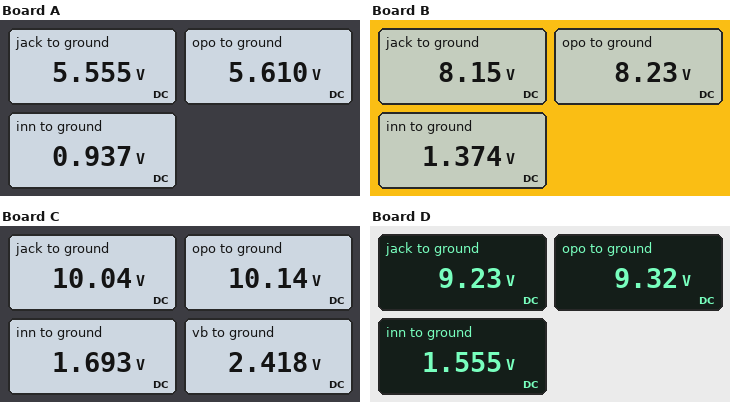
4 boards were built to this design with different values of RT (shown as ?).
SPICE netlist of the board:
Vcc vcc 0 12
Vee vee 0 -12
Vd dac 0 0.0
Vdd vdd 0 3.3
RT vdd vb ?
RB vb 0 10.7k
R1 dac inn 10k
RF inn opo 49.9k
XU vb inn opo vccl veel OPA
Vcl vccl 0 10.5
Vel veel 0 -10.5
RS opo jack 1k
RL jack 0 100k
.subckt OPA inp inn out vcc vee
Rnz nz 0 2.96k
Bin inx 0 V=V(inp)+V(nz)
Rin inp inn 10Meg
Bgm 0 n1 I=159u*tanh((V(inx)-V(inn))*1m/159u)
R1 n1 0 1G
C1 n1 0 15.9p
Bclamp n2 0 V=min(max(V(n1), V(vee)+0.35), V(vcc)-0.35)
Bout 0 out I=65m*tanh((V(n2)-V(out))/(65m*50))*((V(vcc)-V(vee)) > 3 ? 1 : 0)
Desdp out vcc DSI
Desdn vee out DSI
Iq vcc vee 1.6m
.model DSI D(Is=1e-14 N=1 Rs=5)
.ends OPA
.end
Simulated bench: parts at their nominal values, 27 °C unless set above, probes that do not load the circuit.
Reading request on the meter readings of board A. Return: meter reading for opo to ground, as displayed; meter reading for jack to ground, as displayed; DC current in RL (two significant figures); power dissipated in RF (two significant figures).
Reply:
5.610 V
5.555 V
56 µA
440 µW
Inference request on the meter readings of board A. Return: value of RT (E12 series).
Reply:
27 kΩ
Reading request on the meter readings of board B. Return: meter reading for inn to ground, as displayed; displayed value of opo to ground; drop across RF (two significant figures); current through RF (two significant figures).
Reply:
1.374 V
8.23 V
6.9 V
140 µA
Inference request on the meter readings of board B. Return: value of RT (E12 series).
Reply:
15 kΩ
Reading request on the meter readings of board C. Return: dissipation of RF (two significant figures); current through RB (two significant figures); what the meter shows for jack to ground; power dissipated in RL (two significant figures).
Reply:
1.4 mW
230 µA
10.04 V
1.0 mW
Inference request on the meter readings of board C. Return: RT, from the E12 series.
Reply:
3.9 kΩ
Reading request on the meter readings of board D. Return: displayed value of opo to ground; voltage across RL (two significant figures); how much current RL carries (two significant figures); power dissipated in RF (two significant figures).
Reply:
9.32 V
9.2 V
92 µA
1.2 mW
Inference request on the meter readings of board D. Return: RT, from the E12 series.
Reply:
12 kΩ
